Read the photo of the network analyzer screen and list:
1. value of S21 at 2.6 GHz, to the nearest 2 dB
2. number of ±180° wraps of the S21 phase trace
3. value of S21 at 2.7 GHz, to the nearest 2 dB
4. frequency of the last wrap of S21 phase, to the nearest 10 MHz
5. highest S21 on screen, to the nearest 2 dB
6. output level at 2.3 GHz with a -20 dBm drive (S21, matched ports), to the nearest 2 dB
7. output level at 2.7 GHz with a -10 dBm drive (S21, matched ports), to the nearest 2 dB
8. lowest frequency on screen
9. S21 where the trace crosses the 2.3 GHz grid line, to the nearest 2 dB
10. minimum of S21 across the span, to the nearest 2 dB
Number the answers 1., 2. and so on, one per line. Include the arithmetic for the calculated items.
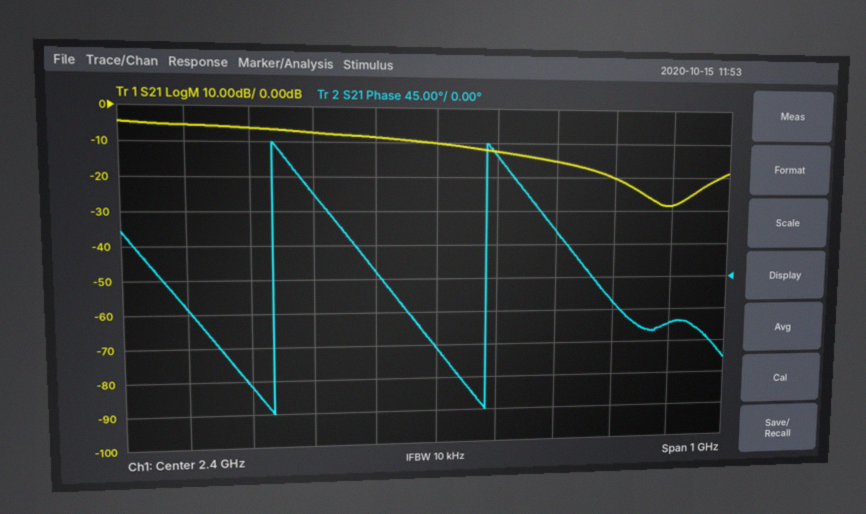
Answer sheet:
1. -16 dB
2. 2
3. -20 dB
4. 2.48 GHz
5. -4 dB
6. -20 dBm + (-8 dB) = -28 dBm
7. -10 dBm + (-20 dB) = -30 dBm
8. 1.9 GHz
9. -8 dB
10. -28 dB
